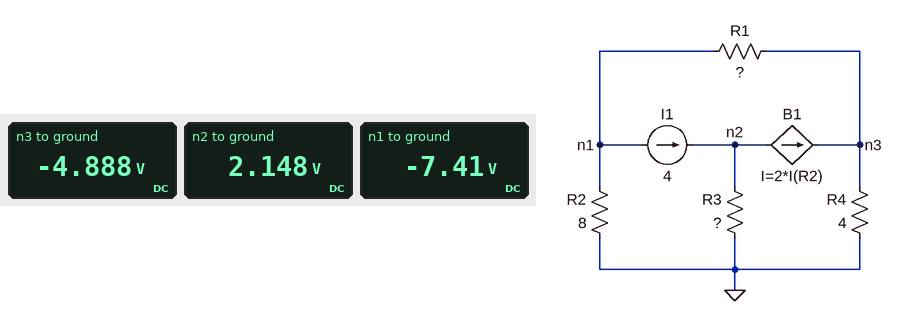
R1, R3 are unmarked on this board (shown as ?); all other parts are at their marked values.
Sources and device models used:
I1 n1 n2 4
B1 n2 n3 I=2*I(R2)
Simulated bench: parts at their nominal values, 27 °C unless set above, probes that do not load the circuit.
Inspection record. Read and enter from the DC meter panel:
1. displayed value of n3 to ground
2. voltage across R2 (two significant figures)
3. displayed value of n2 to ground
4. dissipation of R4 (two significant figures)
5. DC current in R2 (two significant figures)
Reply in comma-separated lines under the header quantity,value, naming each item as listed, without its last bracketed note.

quantity,value
displayed value of n3 to ground,-4.888 V
voltage across R2,7.4 V
displayed value of n2 to ground,2.148 V
dissipation of R4,6.0 W
DC current in R2,930 mA
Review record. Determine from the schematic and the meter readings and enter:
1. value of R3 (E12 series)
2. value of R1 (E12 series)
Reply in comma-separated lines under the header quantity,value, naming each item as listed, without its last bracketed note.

quantity,value
value of R3,1 Ω
value of R1,0.82 Ω
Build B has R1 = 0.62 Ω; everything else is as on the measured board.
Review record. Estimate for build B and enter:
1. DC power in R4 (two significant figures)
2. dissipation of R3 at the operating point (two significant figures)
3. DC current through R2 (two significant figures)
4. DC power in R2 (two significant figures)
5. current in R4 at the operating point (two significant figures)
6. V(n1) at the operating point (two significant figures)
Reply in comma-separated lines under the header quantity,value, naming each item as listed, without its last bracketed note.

quantity,value
DC power in R4,6.9 W
dissipation of R3 at the operating point,4.9 W
DC current through R2,900 mA
DC power in R2,6.4 W
current in R4 at the operating point,1.3 A
V(n1) at the operating point,-7.2 V
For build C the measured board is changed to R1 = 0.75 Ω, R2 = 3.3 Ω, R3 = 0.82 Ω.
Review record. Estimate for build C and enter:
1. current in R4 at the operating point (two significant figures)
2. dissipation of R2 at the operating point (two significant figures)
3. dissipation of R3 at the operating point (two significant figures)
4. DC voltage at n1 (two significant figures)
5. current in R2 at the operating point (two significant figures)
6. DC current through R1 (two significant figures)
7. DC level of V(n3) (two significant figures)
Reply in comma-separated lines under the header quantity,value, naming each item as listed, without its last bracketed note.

quantity,value
current in R4 at the operating point,450 mA
dissipation of R2 at the operating point,4.6 W
dissipation of R3 at the operating point,2.2 W
DC voltage at n1,-3.9 V
current in R2 at the operating point,1.2 A
DC current through R1,2.8 A
DC level of V(n3),-1.8 V
